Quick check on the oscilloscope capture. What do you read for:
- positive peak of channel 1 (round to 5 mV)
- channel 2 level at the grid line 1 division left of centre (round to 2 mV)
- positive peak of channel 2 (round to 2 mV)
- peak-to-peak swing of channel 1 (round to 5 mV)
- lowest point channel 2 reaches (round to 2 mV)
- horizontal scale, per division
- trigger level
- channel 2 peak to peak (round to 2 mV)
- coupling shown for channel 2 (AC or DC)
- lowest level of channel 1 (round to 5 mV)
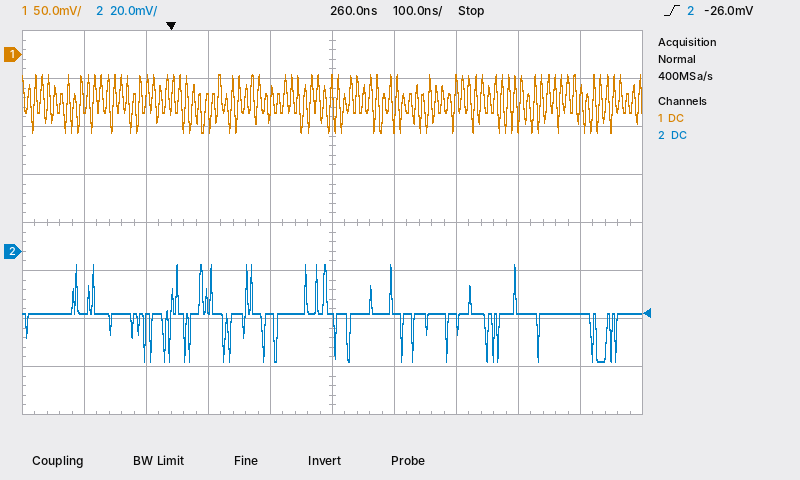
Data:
-20 mV
-26 mV
-6 mV
60 mV
-46 mV
100 ns
-26.0 mV
40 mV
DC
-80 mV
